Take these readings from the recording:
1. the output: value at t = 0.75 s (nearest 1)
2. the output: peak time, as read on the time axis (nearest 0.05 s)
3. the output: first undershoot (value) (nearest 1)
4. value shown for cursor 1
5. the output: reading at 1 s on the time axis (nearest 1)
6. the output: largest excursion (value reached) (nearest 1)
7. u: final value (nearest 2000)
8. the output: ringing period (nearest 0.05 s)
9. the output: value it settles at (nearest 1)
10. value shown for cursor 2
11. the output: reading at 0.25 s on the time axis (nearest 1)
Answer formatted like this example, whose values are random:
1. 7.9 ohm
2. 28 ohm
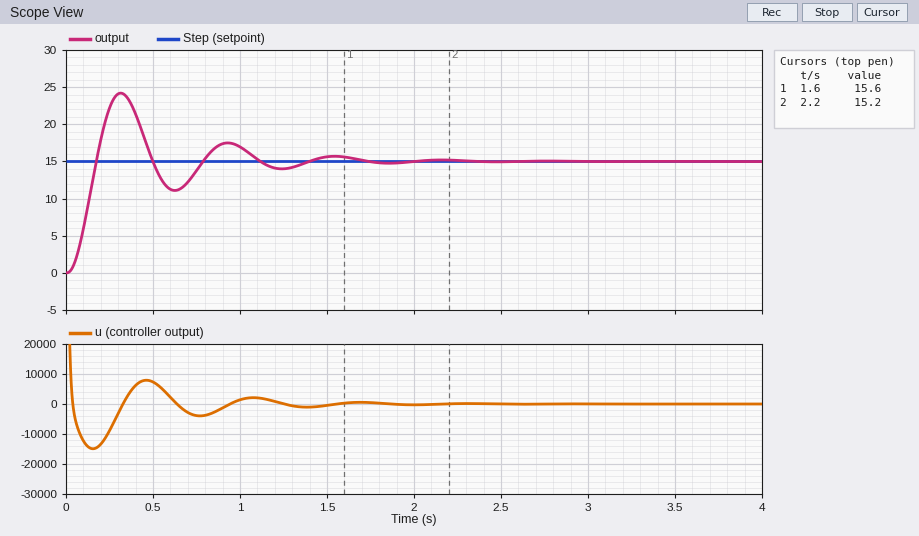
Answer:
1. 14
2. 0.30 s
3. 11
4. 15.6
5. 17
6. 24
7. 0
8. 0.60 s
9. 15
10. 15.2
11. 22
